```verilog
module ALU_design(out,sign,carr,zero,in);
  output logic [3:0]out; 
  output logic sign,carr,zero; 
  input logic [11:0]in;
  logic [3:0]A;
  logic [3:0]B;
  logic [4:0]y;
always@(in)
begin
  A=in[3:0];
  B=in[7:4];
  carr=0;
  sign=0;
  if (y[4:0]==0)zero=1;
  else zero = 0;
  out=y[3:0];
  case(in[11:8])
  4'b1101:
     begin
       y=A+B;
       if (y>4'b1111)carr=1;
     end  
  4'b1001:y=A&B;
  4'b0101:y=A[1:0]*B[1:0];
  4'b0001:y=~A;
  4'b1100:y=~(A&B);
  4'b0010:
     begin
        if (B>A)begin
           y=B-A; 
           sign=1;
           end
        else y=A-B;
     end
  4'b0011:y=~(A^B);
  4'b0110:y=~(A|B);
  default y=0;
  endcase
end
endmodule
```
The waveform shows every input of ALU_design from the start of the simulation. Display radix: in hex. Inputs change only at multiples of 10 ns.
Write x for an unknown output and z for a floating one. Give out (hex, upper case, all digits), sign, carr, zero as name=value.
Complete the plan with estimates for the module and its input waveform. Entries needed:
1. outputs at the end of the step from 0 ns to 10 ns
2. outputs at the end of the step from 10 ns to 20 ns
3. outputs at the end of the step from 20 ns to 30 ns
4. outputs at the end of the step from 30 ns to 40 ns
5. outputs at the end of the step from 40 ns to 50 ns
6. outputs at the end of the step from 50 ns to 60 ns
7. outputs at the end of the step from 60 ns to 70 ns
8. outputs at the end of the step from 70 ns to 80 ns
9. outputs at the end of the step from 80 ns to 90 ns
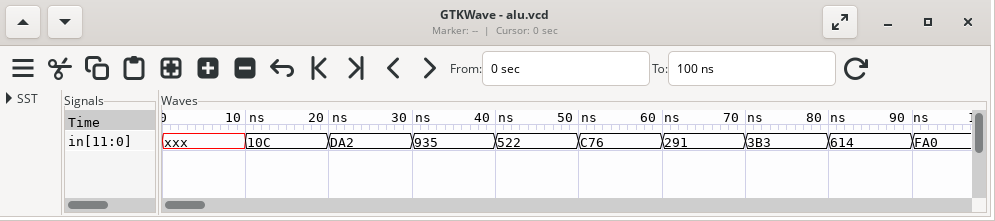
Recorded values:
out=x, sign=x, carr=x, zero=x
out=x, sign=0, carr=0, zero=0
out=3, sign=0, carr=0, zero=0
out=C, sign=0, carr=0, zero=0
out=1, sign=0, carr=0, zero=0
out=4, sign=0, carr=0, zero=0
out=9, sign=1, carr=0, zero=0
out=8, sign=0, carr=0, zero=0
out=7, sign=0, carr=0, zero=0
